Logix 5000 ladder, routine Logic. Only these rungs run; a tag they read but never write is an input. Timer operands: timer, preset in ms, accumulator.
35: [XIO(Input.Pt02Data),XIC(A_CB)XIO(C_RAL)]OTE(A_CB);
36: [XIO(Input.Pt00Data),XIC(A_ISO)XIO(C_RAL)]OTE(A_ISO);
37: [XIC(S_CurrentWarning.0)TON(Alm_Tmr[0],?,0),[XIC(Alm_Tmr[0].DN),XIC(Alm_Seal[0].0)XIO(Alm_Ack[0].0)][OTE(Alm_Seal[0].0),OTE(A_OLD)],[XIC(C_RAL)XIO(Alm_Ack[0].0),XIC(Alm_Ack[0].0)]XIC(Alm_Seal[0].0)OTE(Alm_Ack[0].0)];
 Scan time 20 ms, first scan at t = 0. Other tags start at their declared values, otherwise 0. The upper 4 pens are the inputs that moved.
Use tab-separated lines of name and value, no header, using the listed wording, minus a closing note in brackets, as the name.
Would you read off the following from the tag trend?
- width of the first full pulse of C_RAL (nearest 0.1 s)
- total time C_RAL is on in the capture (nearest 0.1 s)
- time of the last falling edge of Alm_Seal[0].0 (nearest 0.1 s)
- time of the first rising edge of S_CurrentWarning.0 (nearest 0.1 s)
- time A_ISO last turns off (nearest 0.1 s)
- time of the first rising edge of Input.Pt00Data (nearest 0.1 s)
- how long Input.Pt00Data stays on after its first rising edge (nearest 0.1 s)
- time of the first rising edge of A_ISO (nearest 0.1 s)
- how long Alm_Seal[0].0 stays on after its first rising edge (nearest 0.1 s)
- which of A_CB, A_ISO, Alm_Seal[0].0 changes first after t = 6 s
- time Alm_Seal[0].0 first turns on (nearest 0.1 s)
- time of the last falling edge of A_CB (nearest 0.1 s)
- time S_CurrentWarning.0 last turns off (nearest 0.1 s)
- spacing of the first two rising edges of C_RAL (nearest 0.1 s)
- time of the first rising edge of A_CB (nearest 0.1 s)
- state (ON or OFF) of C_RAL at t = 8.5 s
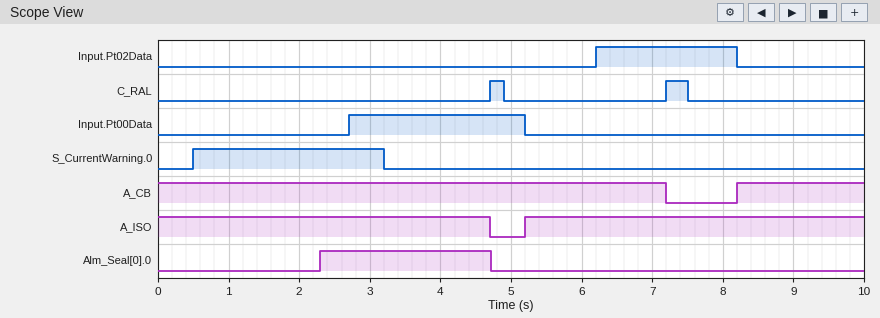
width of the first full pulse of C_RAL	0.2 s
total time C_RAL is on in the capture	0.5 s
time of the last falling edge of Alm_Seal[0].0	4.7 s
time of the first rising edge of S_CurrentWarning.0	0.5 s
time A_ISO last turns off	4.7 s
time of the first rising edge of Input.Pt00Data	2.7 s
how long Input.Pt00Data stays on after its first rising edge	2.5 s
time of the first rising edge of A_ISO	5.2 s
how long Alm_Seal[0].0 stays on after its first rising edge	2.4 s
which of A_CB, A_ISO, Alm_Seal[0].0 changes first after t = 6 s	A_CB
time Alm_Seal[0].0 first turns on	2.3 s
time of the last falling edge of A_CB	7.2 s
time S_CurrentWarning.0 last turns off	3.2 s
spacing of the first two rising edges of C_RAL	2.5 s
time of the first rising edge of A_CB	8.2 s
state (ON or OFF) of C_RAL at t = 8.5 s	OFF
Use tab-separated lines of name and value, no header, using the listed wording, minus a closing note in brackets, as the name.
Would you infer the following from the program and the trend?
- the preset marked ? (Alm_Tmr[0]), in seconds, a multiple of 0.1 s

the preset marked ? (Alm_Tmr[0]), in seconds, a multiple of 0.1 s	1.8 s
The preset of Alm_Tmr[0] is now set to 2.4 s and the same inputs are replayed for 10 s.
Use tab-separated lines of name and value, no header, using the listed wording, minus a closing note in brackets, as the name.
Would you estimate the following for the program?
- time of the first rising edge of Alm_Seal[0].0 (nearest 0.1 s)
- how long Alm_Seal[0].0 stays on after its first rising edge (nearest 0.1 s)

time of the first rising edge of Alm_Seal[0].0	2.9 s
how long Alm_Seal[0].0 stays on after its first rising edge	1.8 s
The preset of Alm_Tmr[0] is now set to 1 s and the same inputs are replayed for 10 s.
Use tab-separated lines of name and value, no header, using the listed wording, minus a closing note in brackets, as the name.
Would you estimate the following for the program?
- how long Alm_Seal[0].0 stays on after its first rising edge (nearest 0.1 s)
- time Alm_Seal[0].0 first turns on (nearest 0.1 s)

how long Alm_Seal[0].0 stays on after its first rising edge	3.2 s
time Alm_Seal[0].0 first turns on	1.5 s
